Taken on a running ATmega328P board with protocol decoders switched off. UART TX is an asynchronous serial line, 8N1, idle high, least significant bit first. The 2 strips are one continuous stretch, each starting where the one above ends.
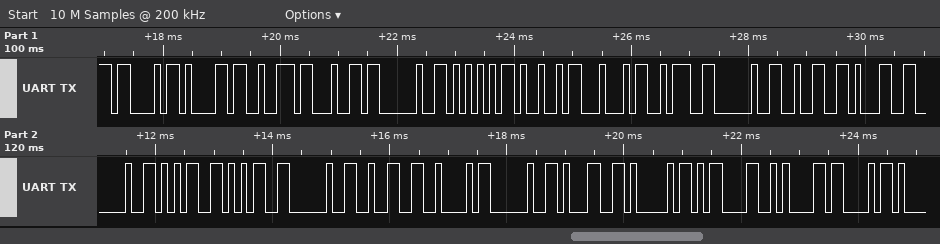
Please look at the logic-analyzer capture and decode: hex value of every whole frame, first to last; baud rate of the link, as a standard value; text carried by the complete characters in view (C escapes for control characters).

43 61 72 64 20 55 49 44 3A 20 32 31 20 35 35 20 32 42 20 31 41 0D 0A 43
9600 baud
"Card UID: 21 55 2B 1A\r\nC"
